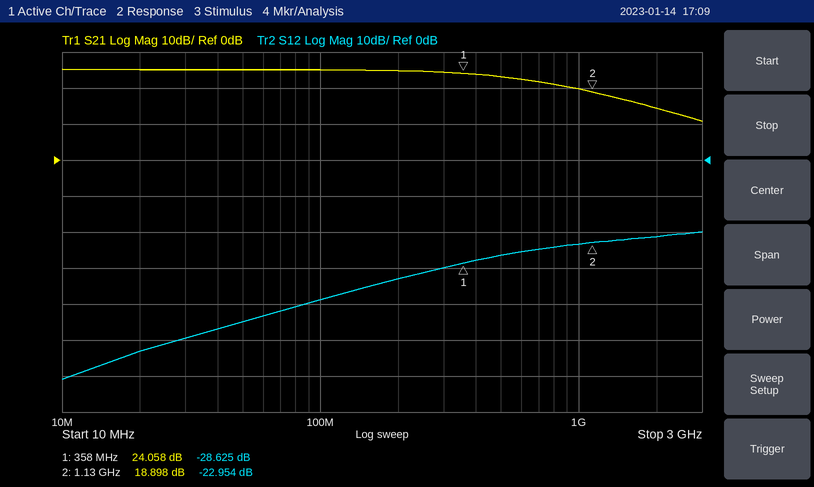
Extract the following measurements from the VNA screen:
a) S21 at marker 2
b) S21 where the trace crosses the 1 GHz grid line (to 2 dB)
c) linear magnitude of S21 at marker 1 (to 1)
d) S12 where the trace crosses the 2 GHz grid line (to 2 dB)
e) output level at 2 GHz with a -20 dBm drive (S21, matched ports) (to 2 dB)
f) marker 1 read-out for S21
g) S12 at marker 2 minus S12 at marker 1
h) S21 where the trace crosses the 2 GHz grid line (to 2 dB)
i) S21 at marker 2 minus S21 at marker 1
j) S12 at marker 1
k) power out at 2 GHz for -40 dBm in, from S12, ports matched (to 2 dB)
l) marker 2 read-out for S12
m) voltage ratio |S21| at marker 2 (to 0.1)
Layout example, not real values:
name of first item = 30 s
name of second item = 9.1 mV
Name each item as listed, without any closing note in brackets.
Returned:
S21 at marker 2 = 18.898 dB
S21 where the trace crosses the 1 GHz grid line = 20 dB
linear magnitude of S21 at marker 1 = 16
S12 where the trace crosses the 2 GHz grid line = -22 dB
output level at 2 GHz with a -20 dBm drive (S21, matched ports) = -6 dBm
marker 1 read-out for S21 = 24.058 dB
S12 at marker 2 minus S12 at marker 1 = 5.671 dB
S21 where the trace crosses the 2 GHz grid line = 14 dB
S21 at marker 2 minus S21 at marker 1 = -5.160 dB
S12 at marker 1 = -28.625 dB
power out at 2 GHz for -40 dBm in, from S12, ports matched = -62 dBm
marker 2 read-out for S12 = -22.954 dB
voltage ratio |S21| at marker 2 = 8.8
